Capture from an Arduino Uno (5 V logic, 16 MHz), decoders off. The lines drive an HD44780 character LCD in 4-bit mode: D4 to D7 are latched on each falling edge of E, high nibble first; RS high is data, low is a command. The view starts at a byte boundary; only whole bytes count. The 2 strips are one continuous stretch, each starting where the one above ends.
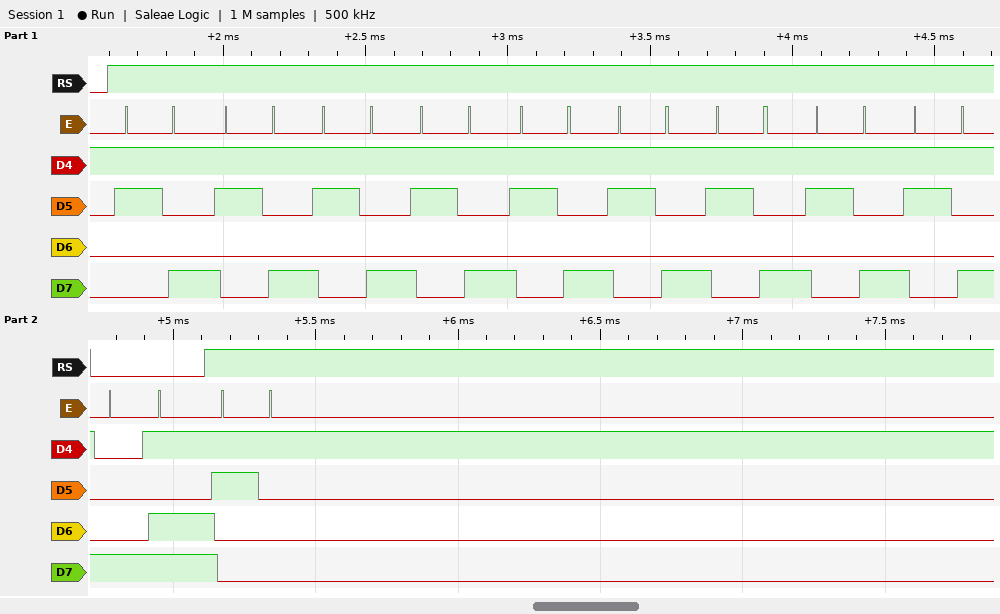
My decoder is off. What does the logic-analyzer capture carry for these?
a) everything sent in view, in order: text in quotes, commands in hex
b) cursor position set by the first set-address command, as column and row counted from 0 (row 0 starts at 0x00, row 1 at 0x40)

"999999999" 0x8D "1"
column 13, row 0
